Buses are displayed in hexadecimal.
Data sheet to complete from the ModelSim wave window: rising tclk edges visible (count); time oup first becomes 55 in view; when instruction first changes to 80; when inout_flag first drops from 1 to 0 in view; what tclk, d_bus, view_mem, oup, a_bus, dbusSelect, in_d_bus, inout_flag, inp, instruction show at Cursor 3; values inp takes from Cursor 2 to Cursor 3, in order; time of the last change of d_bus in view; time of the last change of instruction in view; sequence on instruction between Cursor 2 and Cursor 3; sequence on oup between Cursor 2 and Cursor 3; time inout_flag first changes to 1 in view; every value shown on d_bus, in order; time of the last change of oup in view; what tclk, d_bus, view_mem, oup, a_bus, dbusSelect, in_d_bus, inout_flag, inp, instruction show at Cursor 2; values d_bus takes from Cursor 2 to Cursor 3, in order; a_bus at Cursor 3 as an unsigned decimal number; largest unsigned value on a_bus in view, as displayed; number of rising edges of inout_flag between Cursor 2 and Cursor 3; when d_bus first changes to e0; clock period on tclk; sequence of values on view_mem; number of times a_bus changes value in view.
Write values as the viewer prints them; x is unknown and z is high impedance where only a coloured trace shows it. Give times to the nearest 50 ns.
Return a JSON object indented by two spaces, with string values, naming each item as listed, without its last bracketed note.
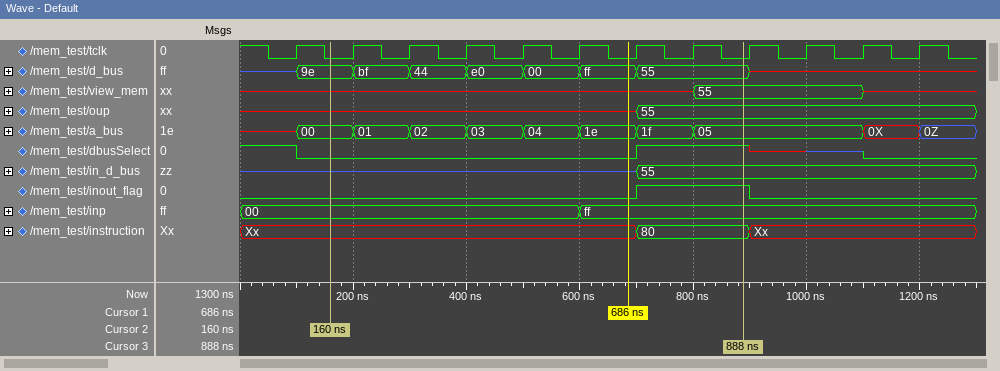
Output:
{
  "rising tclk edges visible": "12",
  "time oup first becomes 55 in view": "700 ns",
  "when instruction first changes to 80": "700 ns",
  "when inout_flag first drops from 1 to 0 in view": "900 ns",
  "what tclk, d_bus, view_mem, oup, a_bus, dbusSelect, in_d_bus, inout_flag, inp, instruction show at Cursor 3": "tclk=0, d_bus=55, view_mem=55, oup=55, a_bus=05, dbusSelect=1, in_d_bus=55, inout_flag=1, inp=ff, instruction=80",
  "values inp takes from Cursor 2 to Cursor 3, in order": "00, ff",
  "time of the last change of d_bus in view": "900 ns",
  "time of the last change of instruction in view": "900 ns",
  "sequence on instruction between Cursor 2 and Cursor 3": "Xx, 80",
  "sequence on oup between Cursor 2 and Cursor 3": "x, 55",
  "time inout_flag first changes to 1 in view": "700 ns",
  "every value shown on d_bus, in order": "z, 9e, bf, 44, e0, 00, ff, 55, x",
  "time of the last change of oup in view": "700 ns",
  "what tclk, d_bus, view_mem, oup, a_bus, dbusSelect, in_d_bus, inout_flag, inp, instruction show at Cursor 2": "tclk=0, d_bus=9e, view_mem=x, oup=x, a_bus=00, dbusSelect=0, in_d_bus=z, inout_flag=0, inp=00, instruction=Xx",
  "values d_bus takes from Cursor 2 to Cursor 3, in order": "9e, bf, 44, e0, 00, ff, 55",
  "a_bus at Cursor 3 as an unsigned decimal number": "5",
  "largest unsigned value on a_bus in view, as displayed": "1f",
  "number of rising edges of inout_flag between Cursor 2 and Cursor 3": "1",
  "when d_bus first changes to e0": "400 ns",
  "clock period on tclk": "100 ns",
  "sequence of values on view_mem": "x, 55, x",
  "number of times a_bus changes value in view": "10"
}
